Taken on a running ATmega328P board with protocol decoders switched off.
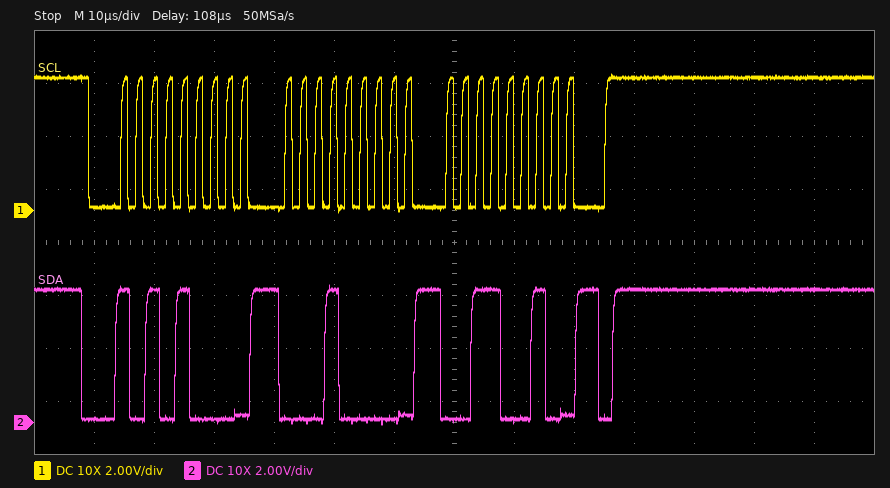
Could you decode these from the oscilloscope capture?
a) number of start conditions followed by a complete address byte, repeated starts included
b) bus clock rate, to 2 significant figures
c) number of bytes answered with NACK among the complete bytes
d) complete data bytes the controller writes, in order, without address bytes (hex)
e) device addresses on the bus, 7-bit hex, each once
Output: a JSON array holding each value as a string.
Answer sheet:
["1", "400 kHz", "0", "10 32", "0x54"]
